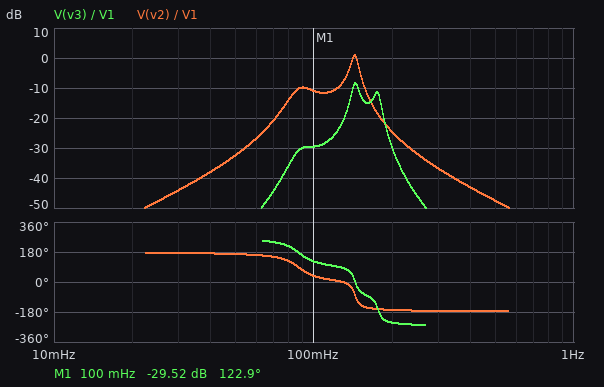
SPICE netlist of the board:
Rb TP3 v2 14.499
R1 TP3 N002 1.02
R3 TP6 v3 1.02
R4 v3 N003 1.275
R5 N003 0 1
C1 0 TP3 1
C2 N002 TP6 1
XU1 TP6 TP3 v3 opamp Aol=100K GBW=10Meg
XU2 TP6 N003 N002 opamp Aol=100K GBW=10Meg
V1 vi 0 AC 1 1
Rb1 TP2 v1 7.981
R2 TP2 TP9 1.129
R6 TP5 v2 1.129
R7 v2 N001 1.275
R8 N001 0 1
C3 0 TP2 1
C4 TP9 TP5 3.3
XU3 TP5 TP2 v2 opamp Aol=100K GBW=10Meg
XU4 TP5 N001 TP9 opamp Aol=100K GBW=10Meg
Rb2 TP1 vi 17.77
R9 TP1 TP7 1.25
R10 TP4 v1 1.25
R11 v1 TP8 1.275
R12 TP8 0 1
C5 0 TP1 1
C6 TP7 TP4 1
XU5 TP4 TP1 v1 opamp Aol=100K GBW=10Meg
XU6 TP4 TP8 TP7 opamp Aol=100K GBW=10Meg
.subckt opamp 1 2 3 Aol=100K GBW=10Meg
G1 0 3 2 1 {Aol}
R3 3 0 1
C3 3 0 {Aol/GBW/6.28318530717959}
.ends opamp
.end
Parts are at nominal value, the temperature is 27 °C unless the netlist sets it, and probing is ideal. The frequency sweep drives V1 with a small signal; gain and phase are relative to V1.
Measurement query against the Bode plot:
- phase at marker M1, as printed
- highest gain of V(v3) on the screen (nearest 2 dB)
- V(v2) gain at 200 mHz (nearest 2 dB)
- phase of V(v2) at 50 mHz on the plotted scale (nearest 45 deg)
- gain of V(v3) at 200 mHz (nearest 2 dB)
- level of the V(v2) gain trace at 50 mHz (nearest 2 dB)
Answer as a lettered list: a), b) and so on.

a) 122.9 deg
b) -8 dB
c) -24 dB
d) 180 deg
e) -30 dB
f) -32 dB
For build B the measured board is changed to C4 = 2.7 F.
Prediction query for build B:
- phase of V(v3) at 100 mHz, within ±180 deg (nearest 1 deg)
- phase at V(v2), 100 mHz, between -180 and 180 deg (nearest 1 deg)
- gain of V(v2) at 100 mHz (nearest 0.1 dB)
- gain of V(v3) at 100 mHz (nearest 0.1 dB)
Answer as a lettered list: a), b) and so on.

a) 155 deg
b) 68 deg
c) -7.7 dB
d) -26.2 dB
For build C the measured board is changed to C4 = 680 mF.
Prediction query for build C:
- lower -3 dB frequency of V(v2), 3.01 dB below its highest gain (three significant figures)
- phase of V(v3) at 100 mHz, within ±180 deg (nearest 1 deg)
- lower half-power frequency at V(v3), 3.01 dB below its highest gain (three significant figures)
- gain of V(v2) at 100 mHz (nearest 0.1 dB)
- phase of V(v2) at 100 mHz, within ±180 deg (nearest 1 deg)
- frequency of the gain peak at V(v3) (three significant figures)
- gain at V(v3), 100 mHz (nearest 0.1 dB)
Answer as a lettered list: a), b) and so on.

a) 140 mHz
b) -102 deg
c) 172 mHz
d) -30.0 dB
e) 171 deg
f) 177 mHz
g) -48.5 dB
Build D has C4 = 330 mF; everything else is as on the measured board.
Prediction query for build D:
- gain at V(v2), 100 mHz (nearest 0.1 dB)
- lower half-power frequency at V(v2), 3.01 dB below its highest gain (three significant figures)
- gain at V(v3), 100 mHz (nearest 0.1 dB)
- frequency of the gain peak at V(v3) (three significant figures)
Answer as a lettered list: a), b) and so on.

a) -37.8 dB
b) 140 mHz
c) -56.3 dB
d) 176 mHz
